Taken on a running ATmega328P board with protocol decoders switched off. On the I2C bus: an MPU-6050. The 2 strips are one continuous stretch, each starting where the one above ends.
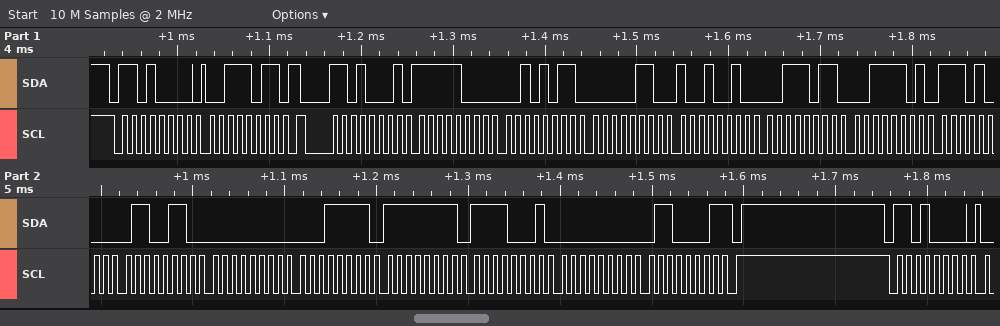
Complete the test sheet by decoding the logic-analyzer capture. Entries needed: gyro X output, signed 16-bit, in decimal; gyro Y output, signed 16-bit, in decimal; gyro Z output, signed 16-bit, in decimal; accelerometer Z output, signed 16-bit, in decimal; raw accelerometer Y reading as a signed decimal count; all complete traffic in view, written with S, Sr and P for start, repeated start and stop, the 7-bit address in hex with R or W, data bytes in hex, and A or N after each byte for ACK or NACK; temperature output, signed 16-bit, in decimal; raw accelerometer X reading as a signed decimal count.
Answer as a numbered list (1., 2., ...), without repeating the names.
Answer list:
1. 31
2. -15
3. 97
4. 15165
5. 1682
6. S 68W A 3B A Sr 68R A F8 A 2B A 06 A 92 A 3B A 3D A E8 A 66 A 00 A 1F A FF A F1 A 00 A 61 N P S 68W A
7. -6042
8. -2005
